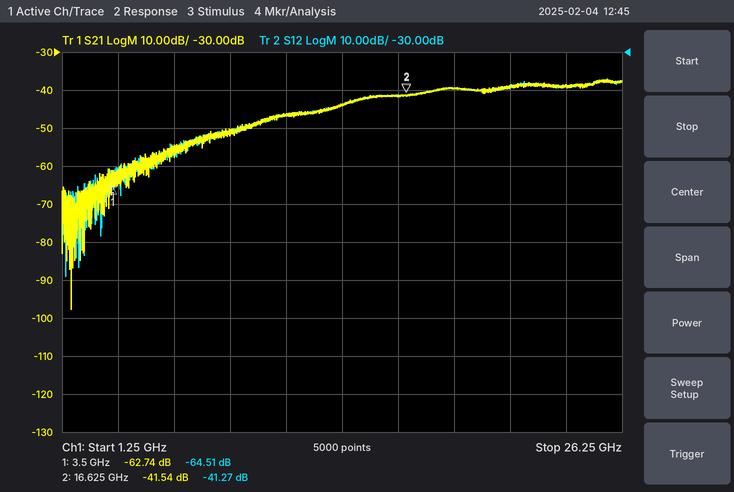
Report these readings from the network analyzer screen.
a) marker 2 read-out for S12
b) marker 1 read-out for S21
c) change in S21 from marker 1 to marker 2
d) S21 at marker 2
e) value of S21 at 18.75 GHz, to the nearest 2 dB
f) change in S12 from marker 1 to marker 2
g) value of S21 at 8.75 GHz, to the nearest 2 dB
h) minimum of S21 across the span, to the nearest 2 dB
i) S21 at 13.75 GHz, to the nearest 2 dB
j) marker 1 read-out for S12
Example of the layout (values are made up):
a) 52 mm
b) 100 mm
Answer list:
a) -41.27 dB
b) -62.74 dB
c) 21.20 dB
d) -41.54 dB
e) -40 dB
f) 23.24 dB
g) -52 dB
h) -98 dB
i) -44 dB
j) -64.51 dB
